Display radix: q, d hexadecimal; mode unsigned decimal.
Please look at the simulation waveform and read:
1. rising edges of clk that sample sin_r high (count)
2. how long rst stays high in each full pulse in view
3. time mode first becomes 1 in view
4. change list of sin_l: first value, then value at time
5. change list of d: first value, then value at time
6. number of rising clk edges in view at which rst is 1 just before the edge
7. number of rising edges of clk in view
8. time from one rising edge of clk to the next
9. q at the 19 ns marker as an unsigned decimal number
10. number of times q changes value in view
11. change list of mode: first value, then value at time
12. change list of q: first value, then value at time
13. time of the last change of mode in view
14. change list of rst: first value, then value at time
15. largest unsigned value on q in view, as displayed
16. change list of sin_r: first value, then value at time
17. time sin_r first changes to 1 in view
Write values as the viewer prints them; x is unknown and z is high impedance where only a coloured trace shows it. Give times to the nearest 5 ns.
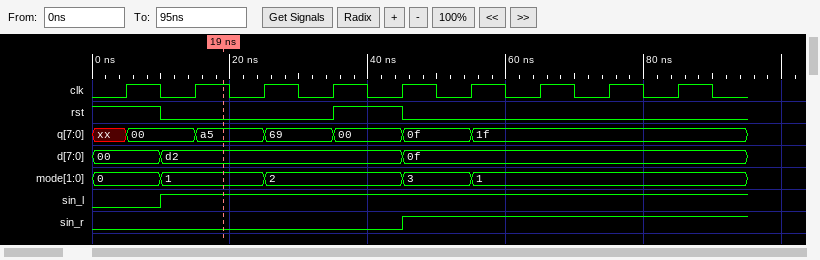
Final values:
4
10 ns
10 ns
0, 1 at 10 ns
00, d2 at 10 ns, 0f at 45 ns
2
9
10 ns
165
6
0, 1 at 10 ns, 2 at 25 ns, 3 at 45 ns, 1 at 55 ns
xx, 00 at 5 ns, a5 at 15 ns, 69 at 25 ns, 00 at 35 ns, 0f at 45 ns, 1f at 55 ns
55 ns
1, 0 at 10 ns, 1 at 35 ns, 0 at 45 ns
a5
0, 1 at 45 ns
45 ns
